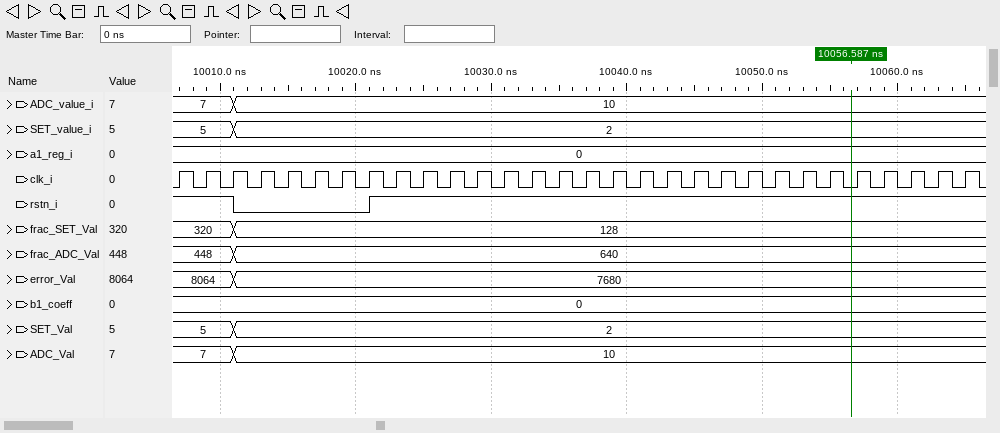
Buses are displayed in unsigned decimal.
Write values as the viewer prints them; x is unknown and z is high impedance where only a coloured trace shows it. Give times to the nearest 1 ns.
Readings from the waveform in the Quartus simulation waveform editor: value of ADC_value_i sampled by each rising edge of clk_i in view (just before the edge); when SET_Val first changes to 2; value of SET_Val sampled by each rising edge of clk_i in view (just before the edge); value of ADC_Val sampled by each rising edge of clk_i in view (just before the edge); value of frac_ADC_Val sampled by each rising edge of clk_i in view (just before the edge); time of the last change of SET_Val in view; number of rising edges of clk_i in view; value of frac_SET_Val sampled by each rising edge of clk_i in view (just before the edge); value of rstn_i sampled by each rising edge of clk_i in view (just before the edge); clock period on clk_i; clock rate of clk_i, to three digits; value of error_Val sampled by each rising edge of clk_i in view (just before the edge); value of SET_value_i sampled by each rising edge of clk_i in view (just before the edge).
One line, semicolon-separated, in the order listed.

7, 7, 7, 10, 10, 10, 10, 10, 10, 10, 10, 10, 10, 10, 10, 10, 10, 10, 10, 10, 10, 10, 10, 10, 10, 10, 10, 10, 10, 10; 10011 ns; 5, 5, 5, 2, 2, 2, 2, 2, 2, 2, 2, 2, 2, 2, 2, 2, 2, 2, 2, 2, 2, 2, 2, 2, 2, 2, 2, 2, 2, 2; 7, 7, 7, 10, 10, 10, 10, 10, 10, 10, 10, 10, 10, 10, 10, 10, 10, 10, 10, 10, 10, 10, 10, 10, 10, 10, 10, 10, 10, 10; 448, 448, 448, 640, 640, 640, 640, 640, 640, 640, 640, 640, 640, 640, 640, 640, 640, 640, 640, 640, 640, 640, 640, 640, 640, 640, 640, 640, 640, 640; 10011 ns; 30; 320, 320, 320, 128, 128, 128, 128, 128, 128, 128, 128, 128, 128, 128, 128, 128, 128, 128, 128, 128, 128, 128, 128, 128, 128, 128, 128, 128, 128, 128; 1 1 1 0 0 0 0 0 1 1 1 1 1 1 1 1 1 1 1 1 1 1 1 1 1 1 1 1 1 1; 2 ns; 500 MHz; 8064, 8064, 8064, 7680, 7680, 7680, 7680, 7680, 7680, 7680, 7680, 7680, 7680, 7680, 7680, 7680, 7680, 7680, 7680, 7680, 7680, 7680, 7680, 7680, 7680, 7680, 7680, 7680, 7680, 7680; 5, 5, 5, 2, 2, 2, 2, 2, 2, 2, 2, 2, 2, 2, 2, 2, 2, 2, 2, 2, 2, 2, 2, 2, 2, 2, 2, 2, 2, 2
